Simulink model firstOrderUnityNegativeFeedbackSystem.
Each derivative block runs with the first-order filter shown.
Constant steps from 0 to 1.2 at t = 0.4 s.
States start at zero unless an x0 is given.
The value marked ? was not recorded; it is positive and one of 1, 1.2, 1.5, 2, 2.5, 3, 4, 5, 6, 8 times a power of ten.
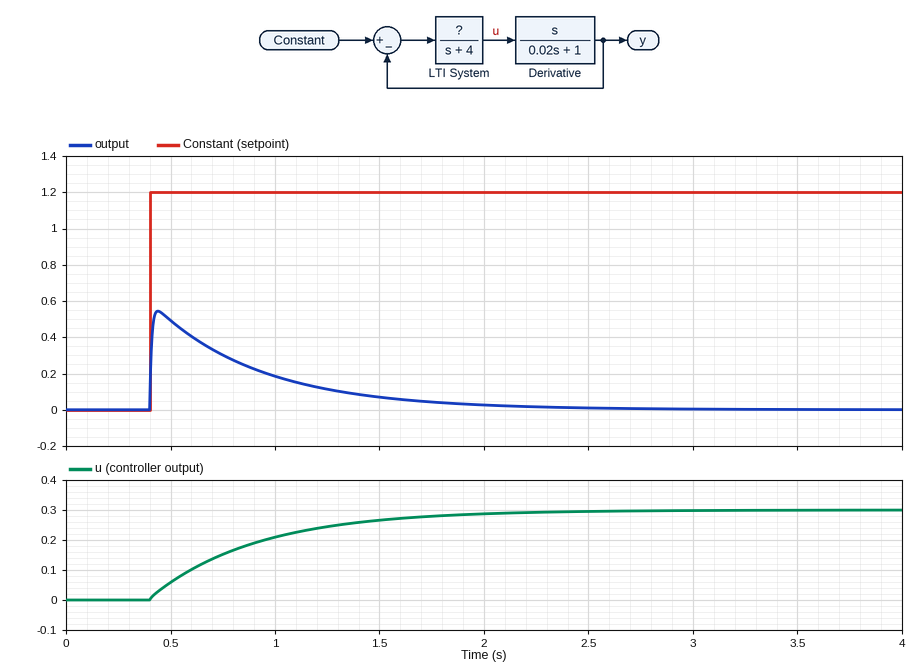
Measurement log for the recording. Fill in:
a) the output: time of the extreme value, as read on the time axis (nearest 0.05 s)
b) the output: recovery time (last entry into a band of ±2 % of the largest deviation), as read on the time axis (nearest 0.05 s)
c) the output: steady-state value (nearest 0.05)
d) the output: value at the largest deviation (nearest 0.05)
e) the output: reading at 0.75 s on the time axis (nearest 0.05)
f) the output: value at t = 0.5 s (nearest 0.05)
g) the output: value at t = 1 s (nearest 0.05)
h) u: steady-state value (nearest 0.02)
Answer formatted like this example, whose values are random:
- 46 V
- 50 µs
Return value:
- 0.45 s
- 2.45 s
- 0.00
- 0.55
- 0.30
- 0.50
- 0.20
- 0.30
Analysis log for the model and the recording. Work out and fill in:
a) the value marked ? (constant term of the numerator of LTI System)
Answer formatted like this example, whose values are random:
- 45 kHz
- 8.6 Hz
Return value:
- 1
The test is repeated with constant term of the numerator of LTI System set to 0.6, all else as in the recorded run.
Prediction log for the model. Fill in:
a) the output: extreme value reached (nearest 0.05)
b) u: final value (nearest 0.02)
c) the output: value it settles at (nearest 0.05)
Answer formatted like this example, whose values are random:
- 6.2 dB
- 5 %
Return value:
- 0.40
- 0.18
- 0.00
